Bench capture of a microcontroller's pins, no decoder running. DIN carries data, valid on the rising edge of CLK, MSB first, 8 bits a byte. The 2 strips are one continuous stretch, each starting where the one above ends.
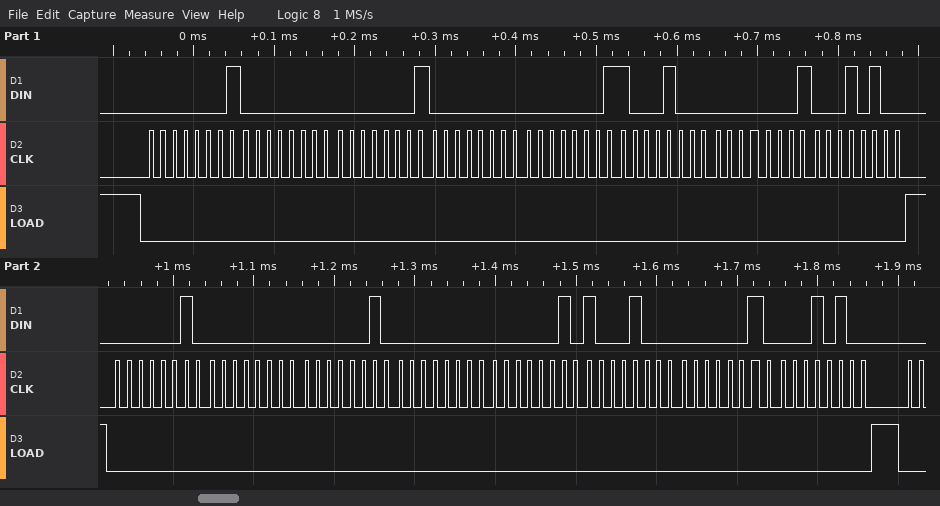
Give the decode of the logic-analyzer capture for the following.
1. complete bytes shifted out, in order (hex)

01 00 01 00 01 88 01 14 02 00 02 00 02 88 02 14
